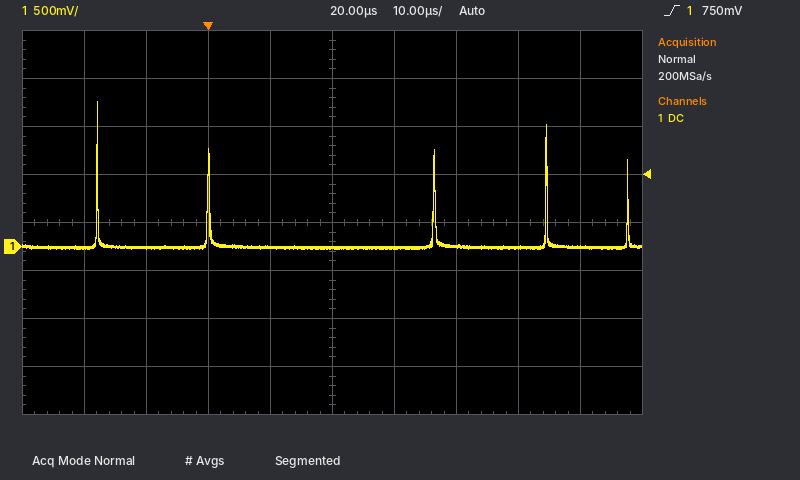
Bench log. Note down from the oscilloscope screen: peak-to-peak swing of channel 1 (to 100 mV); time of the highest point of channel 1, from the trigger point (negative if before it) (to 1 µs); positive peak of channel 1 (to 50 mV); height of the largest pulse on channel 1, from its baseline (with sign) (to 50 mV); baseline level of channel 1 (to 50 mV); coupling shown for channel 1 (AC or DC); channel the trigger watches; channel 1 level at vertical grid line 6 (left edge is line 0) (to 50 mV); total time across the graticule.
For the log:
1.50 V
-18 µs
1.50 V
+1.50 V
0 mV
DC
channel 1
0 mV
100 µs
